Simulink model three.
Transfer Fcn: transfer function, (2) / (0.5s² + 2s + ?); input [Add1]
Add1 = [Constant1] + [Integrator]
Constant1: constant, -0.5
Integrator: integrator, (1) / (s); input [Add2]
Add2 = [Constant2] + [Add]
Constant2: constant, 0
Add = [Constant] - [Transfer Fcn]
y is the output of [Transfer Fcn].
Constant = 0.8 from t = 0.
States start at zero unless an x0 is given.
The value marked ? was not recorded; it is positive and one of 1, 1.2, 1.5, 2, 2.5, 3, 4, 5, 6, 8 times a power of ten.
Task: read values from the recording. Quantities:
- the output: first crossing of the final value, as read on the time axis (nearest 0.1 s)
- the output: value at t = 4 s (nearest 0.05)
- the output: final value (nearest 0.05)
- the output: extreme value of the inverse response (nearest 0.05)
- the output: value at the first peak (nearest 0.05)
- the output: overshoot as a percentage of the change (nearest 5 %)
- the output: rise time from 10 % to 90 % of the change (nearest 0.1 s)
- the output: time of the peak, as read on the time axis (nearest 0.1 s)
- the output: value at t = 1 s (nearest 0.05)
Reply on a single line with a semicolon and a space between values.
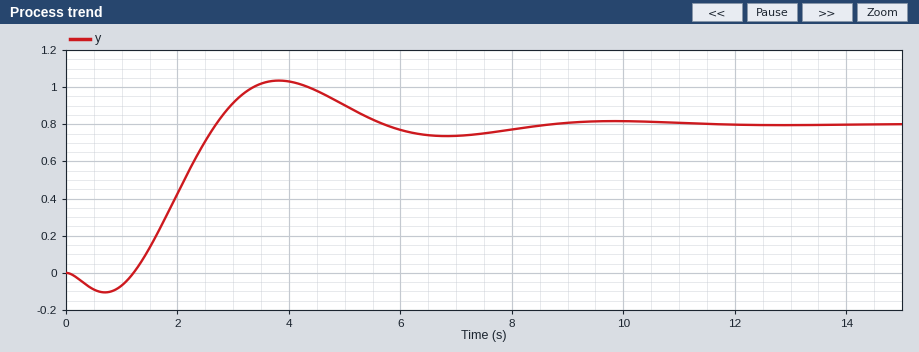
2.7 s; 1.05; 0.80; -0.10; 1.05; 30 %; 1.1 s; 3.8 s; -0.05
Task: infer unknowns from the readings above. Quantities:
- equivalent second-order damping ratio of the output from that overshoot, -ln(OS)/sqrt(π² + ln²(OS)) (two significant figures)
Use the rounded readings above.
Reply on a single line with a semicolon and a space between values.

0.36
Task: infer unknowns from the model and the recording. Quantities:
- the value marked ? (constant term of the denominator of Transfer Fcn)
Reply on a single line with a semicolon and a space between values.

2
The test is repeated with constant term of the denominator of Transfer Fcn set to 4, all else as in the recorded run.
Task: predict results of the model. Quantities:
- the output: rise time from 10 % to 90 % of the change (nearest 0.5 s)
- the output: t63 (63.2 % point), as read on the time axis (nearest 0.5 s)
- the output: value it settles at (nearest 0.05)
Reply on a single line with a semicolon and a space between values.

3.0 s; 2.5 s; 0.80
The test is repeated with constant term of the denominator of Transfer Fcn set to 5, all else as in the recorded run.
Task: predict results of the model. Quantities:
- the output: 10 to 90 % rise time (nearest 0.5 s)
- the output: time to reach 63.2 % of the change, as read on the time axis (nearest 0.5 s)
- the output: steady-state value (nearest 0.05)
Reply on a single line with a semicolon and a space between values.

4.5 s; 3.0 s; 0.80
